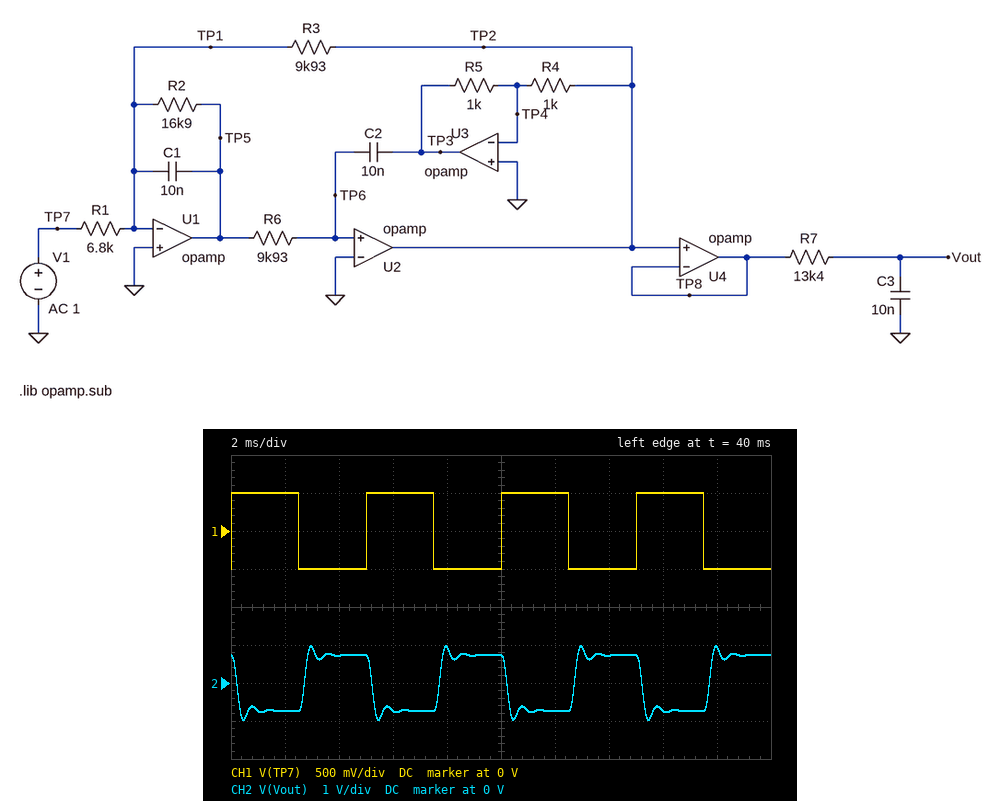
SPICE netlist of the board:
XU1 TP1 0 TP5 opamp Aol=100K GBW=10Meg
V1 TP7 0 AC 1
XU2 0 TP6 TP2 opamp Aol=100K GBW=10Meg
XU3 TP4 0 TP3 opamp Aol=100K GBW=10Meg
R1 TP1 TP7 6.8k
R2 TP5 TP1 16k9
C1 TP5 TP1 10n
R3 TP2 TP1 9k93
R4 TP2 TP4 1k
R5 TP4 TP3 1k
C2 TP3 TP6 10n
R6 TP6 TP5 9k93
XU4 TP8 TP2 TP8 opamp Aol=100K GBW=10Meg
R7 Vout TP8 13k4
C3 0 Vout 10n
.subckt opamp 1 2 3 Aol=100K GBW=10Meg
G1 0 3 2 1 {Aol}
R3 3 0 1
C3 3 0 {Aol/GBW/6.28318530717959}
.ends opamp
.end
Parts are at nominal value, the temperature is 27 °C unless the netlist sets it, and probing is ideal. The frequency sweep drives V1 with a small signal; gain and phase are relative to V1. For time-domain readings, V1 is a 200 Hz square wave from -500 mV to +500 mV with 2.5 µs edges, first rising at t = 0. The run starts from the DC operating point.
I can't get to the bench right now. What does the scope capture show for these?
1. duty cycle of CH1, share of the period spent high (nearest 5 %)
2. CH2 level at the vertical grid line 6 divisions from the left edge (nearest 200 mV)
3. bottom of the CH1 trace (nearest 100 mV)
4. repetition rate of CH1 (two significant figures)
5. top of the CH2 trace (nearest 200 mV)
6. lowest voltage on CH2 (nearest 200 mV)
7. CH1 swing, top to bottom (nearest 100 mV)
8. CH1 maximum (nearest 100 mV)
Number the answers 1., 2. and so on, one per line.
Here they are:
1. 50 %
2. -800 mV
3. -500 mV
4. 200 Hz
5. 1.0 V
6. -1.0 V
7. 1.0 V
8. 500 mV
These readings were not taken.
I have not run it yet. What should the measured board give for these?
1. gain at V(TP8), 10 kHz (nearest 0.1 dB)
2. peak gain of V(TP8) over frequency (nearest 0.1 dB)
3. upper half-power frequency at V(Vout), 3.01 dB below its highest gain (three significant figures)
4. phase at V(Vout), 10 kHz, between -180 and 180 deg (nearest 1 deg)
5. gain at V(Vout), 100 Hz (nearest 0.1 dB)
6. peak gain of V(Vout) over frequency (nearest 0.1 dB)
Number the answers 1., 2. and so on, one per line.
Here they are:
1. -28.3 dB
2. 8.3 dB
3. 1.77 kHz
4. -78 deg
5. 3.3 dB
6. 4.5 dB
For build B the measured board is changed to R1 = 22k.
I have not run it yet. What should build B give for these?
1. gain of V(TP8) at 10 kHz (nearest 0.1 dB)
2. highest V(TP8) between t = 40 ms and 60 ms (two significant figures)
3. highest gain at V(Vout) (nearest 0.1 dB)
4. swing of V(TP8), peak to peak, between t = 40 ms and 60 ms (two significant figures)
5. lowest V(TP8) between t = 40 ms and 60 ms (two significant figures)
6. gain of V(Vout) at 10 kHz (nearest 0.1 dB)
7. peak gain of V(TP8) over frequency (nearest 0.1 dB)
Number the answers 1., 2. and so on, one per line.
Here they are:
1. -38.5 dB
2. 400 mV
3. -5.7 dB
4. 800 mV
5. -400 mV
6. -57.1 dB
7. -1.9 dB
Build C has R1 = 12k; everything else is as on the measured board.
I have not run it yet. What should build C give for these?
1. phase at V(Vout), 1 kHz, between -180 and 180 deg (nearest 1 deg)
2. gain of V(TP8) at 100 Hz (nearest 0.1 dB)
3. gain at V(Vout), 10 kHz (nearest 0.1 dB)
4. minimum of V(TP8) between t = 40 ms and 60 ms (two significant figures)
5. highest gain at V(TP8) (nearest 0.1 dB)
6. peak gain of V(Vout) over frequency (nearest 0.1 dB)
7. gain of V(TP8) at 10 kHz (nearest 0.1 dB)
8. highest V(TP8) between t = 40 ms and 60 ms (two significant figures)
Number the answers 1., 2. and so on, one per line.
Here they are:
1. 109 deg
2. -1.6 dB
3. -51.8 dB
4. -730 mV
5. 3.4 dB
6. -0.4 dB
7. -33.3 dB
8. 730 mV
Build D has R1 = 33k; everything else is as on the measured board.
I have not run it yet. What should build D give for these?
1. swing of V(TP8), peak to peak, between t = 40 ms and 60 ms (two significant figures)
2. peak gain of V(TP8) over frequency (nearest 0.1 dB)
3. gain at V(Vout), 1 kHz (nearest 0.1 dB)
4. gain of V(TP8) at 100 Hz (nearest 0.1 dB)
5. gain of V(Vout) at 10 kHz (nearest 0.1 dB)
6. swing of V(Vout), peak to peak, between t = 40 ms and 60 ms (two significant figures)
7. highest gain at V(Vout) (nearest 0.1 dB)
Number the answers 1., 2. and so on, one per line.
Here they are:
1. 530 mV
2. -5.4 dB
3. -9.8 dB
4. -10.4 dB
5. -60.6 dB
6. 400 mV
7. -9.2 dB
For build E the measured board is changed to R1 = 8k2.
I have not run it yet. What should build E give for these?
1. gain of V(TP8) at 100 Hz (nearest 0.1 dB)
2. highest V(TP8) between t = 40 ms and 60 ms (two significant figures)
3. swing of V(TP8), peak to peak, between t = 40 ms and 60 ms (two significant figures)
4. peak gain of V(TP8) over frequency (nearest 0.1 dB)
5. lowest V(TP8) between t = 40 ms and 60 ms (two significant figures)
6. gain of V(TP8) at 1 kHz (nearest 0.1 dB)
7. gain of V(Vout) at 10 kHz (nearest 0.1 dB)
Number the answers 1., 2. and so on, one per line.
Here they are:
1. 1.7 dB
2. 1.1 V
3. 2.1 V
4. 6.7 dB
5. -1.1 V
6. 4.6 dB
7. -48.5 dB
